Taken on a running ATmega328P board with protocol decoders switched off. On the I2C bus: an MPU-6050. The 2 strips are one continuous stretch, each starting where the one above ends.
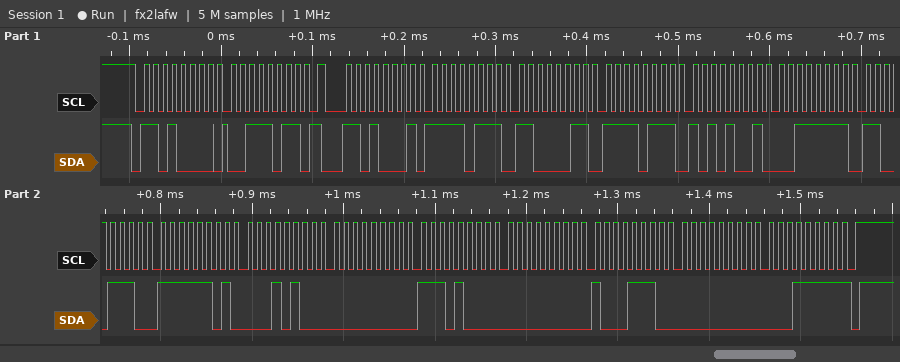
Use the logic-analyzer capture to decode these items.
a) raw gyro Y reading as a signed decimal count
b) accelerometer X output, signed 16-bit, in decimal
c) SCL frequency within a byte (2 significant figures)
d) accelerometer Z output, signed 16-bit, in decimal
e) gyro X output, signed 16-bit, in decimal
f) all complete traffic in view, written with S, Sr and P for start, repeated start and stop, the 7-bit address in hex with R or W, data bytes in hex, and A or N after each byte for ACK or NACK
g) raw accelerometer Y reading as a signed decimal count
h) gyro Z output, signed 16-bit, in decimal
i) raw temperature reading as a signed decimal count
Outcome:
142
-2109
100 kHz
16334
232
S 68W A 3B A Sr 68R A F7 A C3 A F7 A A9 A 3F A CE A FD A 14 A 00 A E8 A 00 A 8E A 00 A 1F N P
-2135
31
-748
